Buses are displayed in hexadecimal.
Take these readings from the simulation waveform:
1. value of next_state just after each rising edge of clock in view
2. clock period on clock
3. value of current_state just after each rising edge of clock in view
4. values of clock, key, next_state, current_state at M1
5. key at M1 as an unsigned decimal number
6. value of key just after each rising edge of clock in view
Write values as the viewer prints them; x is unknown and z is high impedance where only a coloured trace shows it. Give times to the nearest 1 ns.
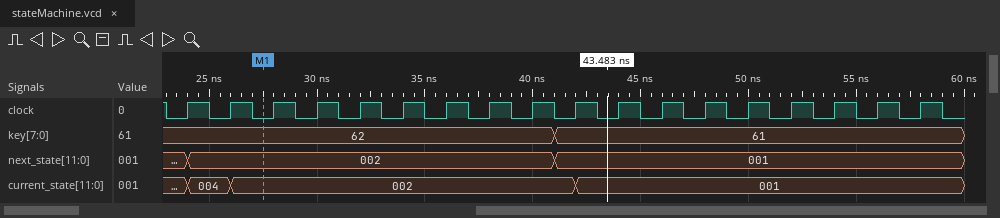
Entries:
002, 002, 002, 002, 002, 002, 002, 002, 002, 001, 001, 001, 001, 001, 001, 001, 001, 001
2 ns
004, 002, 002, 002, 002, 002, 002, 002, 002, 001, 001, 001, 001, 001, 001, 001, 001, 001
clock=0, key=62, next_state=002, current_state=002
98
62, 62, 62, 62, 62, 62, 62, 62, 62, 61, 61, 61, 61, 61, 61, 61, 61, 61
